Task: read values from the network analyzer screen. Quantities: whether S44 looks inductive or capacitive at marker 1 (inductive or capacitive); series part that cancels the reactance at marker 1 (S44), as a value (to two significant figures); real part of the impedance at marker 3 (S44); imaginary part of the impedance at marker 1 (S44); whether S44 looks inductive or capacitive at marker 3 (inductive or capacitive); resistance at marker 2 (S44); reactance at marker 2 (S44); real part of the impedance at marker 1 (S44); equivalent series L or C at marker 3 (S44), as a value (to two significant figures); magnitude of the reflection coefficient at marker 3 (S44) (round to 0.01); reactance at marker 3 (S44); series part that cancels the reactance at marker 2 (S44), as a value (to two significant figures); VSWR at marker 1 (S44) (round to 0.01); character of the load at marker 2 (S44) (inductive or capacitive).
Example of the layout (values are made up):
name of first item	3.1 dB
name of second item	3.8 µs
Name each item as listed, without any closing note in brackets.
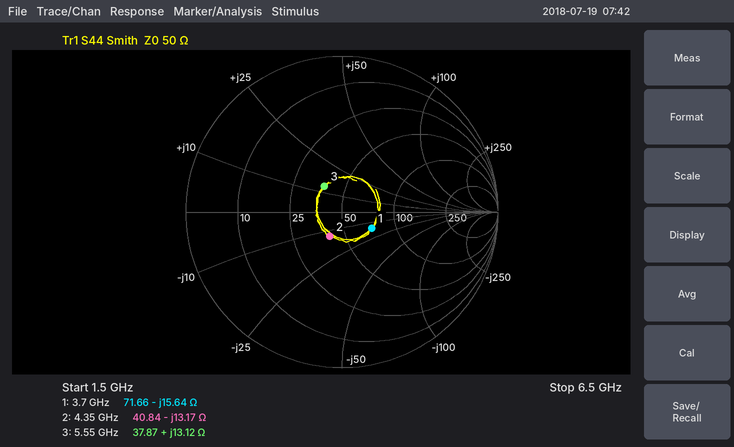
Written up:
whether S44 looks inductive or capacitive at marker 1	capacitive
series part that cancels the reactance at marker 1 (S44), as a value	670 pH
real part of the impedance at marker 3	37.87 Ω
imaginary part of the impedance at marker 1	-15.64 Ω
whether S44 looks inductive or capacitive at marker 3	inductive
resistance at marker 2	40.84 Ω
reactance at marker 2	-13.17 Ω
real part of the impedance at marker 1	71.66 Ω
equivalent series L or C at marker 3 (S44), as a value	380 pH
magnitude of the reflection coefficient at marker 3 (S44)	0.20
reactance at marker 3	+13.12 Ω
series part that cancels the reactance at marker 2 (S44), as a value	480 pH
VSWR at marker 1 (S44)	1.56
character of the load at marker 2 (S44)	capacitive
